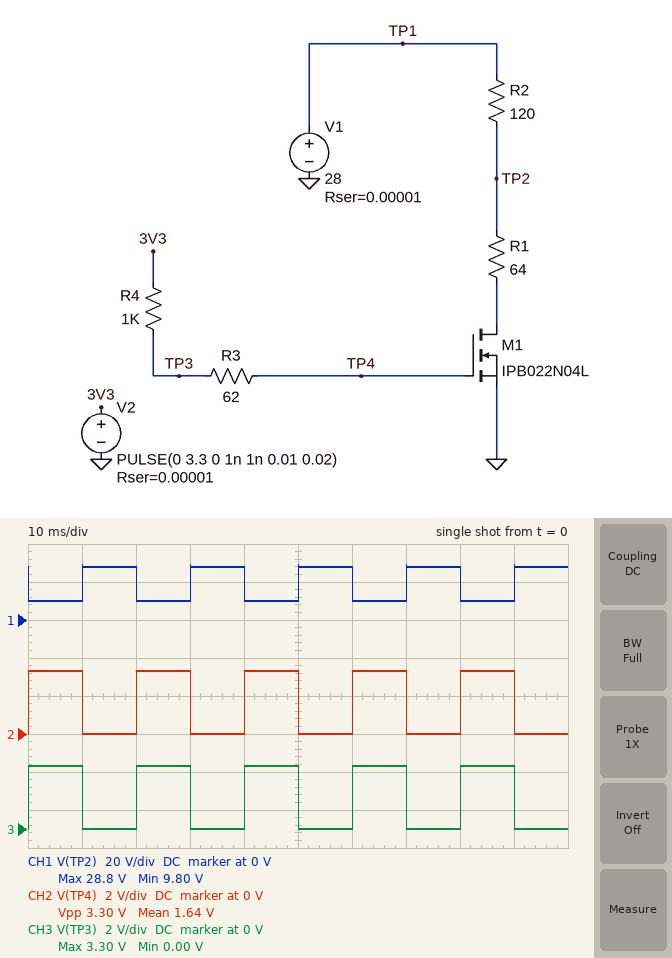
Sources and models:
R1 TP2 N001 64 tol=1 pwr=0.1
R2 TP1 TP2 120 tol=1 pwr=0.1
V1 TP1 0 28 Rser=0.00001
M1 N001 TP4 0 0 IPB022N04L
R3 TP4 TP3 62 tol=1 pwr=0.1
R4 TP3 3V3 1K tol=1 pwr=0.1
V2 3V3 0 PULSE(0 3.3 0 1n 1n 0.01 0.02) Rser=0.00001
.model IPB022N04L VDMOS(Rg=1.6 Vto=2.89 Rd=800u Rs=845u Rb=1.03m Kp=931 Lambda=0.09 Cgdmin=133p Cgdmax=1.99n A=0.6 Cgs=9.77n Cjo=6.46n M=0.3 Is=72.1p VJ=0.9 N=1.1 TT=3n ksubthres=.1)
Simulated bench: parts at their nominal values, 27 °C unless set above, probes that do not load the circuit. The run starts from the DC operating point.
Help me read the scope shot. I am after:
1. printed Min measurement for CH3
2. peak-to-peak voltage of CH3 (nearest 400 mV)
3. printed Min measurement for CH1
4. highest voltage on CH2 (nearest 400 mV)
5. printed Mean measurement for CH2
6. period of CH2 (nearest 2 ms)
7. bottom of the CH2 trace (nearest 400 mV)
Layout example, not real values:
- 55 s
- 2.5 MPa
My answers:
- 0.00 V
- 3.2 V
- 9.80 V
- 3.2 V
- 1.64 V
- 20 ms
- 0 V
